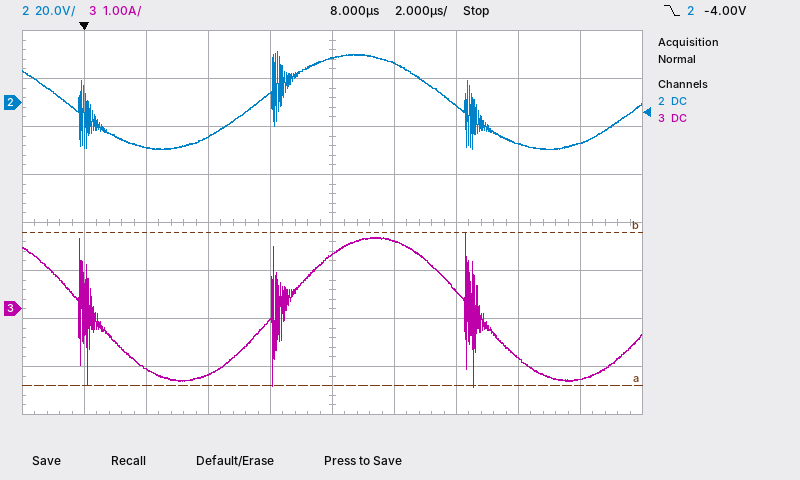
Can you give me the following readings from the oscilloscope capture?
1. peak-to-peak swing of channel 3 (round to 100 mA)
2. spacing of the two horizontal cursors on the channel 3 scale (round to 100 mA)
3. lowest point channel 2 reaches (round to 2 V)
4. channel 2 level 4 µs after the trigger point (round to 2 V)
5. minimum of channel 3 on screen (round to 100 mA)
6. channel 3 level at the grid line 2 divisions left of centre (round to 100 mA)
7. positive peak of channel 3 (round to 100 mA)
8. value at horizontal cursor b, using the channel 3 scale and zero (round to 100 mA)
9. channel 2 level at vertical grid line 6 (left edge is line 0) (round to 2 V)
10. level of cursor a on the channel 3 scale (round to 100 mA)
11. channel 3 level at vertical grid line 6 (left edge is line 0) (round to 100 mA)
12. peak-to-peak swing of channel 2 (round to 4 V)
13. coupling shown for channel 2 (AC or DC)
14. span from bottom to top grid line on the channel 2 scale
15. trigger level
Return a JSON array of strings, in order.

["3.2 A", "3.2 A", "-20 V", "-14 V", "-1.6 A", "-1.4 A", "1.6 A", "1.6 A", "16 V", "-1.6 A", "1.4 A", "40 V", "DC", "160 V", "-4.00 V"]
